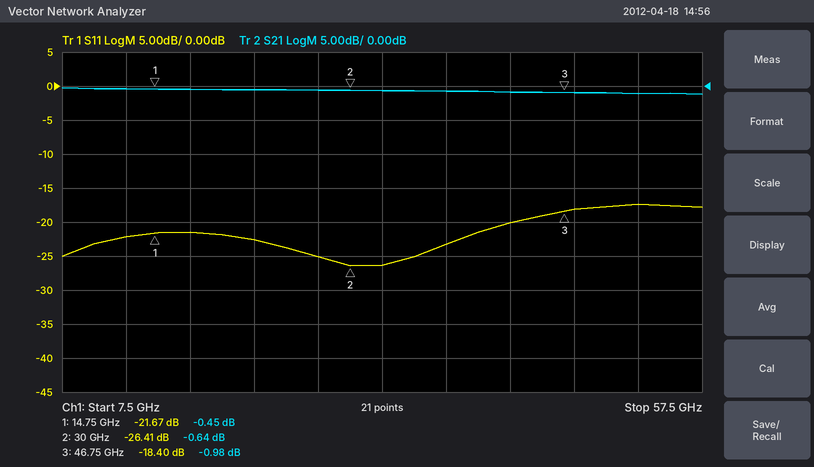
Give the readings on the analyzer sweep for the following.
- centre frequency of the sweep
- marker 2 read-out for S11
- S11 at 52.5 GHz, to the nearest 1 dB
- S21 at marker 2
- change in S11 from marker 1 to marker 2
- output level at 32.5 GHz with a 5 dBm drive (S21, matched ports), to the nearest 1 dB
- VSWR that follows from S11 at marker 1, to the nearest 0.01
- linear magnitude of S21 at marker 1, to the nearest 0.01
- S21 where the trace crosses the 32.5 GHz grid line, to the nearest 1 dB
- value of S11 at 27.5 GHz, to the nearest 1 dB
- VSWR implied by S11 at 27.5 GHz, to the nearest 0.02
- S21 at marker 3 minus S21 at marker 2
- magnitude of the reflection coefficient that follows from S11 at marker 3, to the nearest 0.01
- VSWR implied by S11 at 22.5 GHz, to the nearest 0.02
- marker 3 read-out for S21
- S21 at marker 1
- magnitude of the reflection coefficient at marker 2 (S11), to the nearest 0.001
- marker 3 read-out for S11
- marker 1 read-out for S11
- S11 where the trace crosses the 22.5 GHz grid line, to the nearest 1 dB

32.5 GHz
-26.41 dB
-17 dB
-0.64 dB
-4.74 dB
4 dBm
1.18
0.95
-1 dB
-25 dB
1.12
-0.34 dB
0.12
1.16
-0.98 dB
-0.45 dB
0.048
-18.40 dB
-21.67 dB
-23 dB
